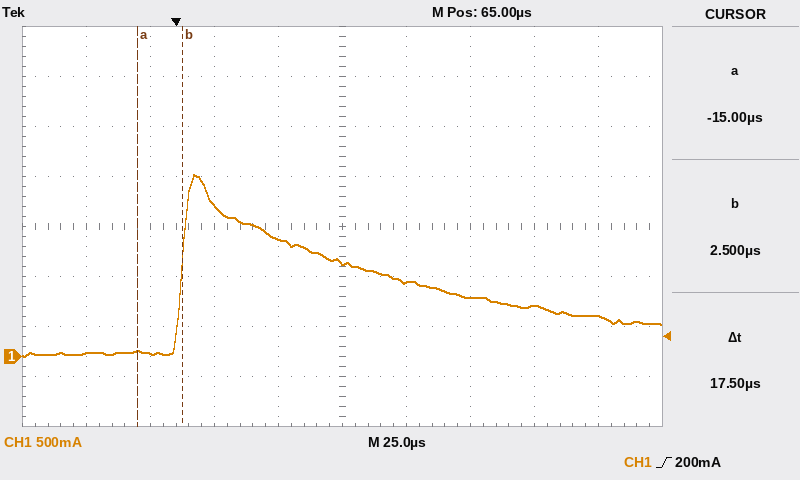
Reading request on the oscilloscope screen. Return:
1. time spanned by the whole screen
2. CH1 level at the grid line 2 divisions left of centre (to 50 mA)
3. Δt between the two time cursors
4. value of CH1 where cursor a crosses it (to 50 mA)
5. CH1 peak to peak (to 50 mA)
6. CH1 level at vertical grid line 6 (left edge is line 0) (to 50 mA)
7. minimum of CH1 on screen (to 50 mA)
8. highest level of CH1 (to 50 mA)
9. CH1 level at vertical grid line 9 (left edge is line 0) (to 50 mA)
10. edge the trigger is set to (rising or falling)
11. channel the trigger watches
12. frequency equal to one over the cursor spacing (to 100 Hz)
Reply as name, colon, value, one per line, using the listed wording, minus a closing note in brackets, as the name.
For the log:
time spanned by the whole screen: 250 µs
CH1 level at the grid line 2 divisions left of centre: 1.50 A
Δt between the two time cursors: 17.5 µs
value of CH1 where cursor a crosses it: 50 mA
CH1 peak to peak: 1.80 A
CH1 level at vertical grid line 6 (left edge is line 0): 750 mA
minimum of CH1 on screen: 0 mA
highest level of CH1: 1.80 A
CH1 level at vertical grid line 9 (left edge is line 0): 400 mA
edge the trigger is set to: rising
channel the trigger watches: CH1
frequency equal to one over the cursor spacing: 57.1 kHz
